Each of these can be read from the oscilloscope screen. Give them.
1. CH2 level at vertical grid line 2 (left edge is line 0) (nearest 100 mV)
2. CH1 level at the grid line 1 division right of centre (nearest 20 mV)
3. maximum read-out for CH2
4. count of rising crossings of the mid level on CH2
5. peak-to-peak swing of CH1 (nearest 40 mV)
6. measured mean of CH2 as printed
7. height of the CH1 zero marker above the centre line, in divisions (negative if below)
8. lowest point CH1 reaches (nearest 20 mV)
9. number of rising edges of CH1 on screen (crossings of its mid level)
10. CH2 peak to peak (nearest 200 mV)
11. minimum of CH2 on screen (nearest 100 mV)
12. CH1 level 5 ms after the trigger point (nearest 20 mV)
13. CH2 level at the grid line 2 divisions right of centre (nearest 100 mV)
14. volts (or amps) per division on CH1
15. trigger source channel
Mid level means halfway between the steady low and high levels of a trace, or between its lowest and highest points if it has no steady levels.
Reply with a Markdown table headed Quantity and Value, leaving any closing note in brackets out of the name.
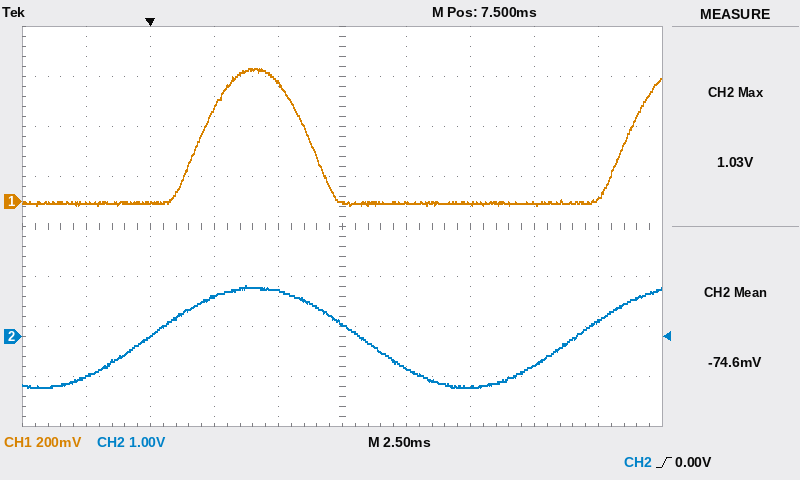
| Quantity | Value |
|---|---|
| CH2 level at vertical grid line 2 (left edge is line 0) | 0.0 V |
| CH1 level at the grid line 1 division right of centre | 0 mV |
| maximum read-out for CH2 | 1.03 V |
| count of rising crossings of the mid level on CH2 | 2 |
| peak-to-peak swing of CH1 | 560 mV |
| measured mean of CH2 as printed | -74.6 mV |
| height of the CH1 zero marker above the centre line, in divisions | +0.5 div |
| lowest point CH1 reaches | -20 mV |
| number of rising edges of CH1 on screen | 2 |
| CH2 peak to peak | 2.0 V |
| minimum of CH2 on screen | -1.0 V |
| CH1 level 5 ms after the trigger point | 480 mV |
| CH2 level at the grid line 2 divisions right of centre | -1.0 V |
| volts (or amps) per division on CH1 | 200 mV |
| trigger source channel | CH2 |
